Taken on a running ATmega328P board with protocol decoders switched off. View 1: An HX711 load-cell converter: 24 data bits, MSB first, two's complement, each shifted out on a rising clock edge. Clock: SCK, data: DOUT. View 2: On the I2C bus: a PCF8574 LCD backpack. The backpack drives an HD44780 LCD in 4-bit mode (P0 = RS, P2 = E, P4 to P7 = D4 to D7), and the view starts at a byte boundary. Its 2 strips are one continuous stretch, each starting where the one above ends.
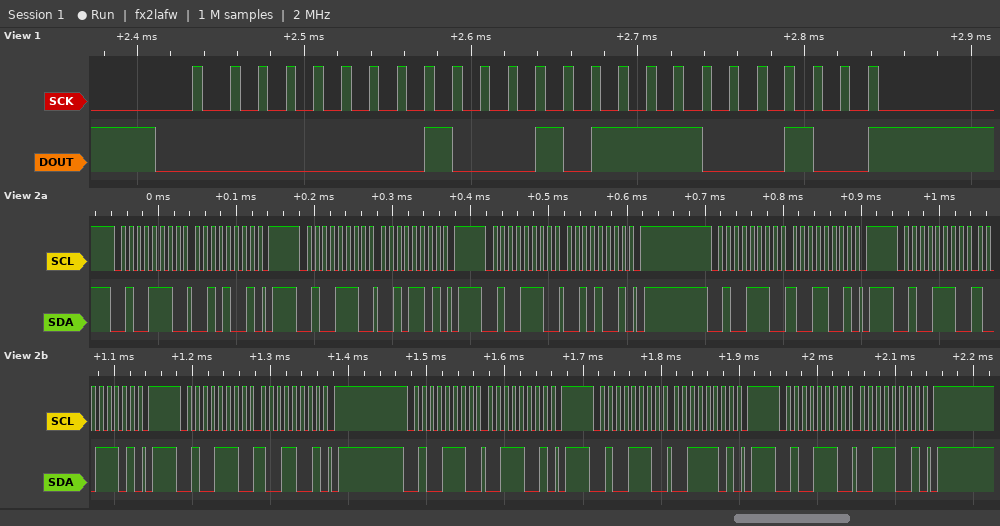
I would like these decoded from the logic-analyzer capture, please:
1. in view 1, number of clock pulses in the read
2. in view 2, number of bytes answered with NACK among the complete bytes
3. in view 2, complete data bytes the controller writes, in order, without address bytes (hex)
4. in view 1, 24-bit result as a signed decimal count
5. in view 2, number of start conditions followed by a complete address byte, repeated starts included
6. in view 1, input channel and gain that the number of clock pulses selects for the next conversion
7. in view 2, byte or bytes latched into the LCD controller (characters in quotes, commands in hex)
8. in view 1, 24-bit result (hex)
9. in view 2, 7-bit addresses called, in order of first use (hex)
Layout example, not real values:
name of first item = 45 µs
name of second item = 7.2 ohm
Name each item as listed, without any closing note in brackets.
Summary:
in view 1, number of clock pulses in the read = 25
in view 2, number of bytes answered with NACK among the complete bytes = 0
in view 2, complete data bytes the controller writes, in order, without address bytes = 29 2D 29 99 9D 99 39 3D 39
in view 1, 24-bit result as a signed decimal count = 35780
in view 2, number of start conditions followed by a complete address byte, repeated starts included = 9
in view 1, input channel and gain that the number of clock pulses selects for the next conversion = channel A, gain 128
in view 2, byte or bytes latched into the LCD controller = ')'
in view 1, 24-bit result = 0x008BC4
in view 2, 7-bit addresses called, in order of first use = 0x27
